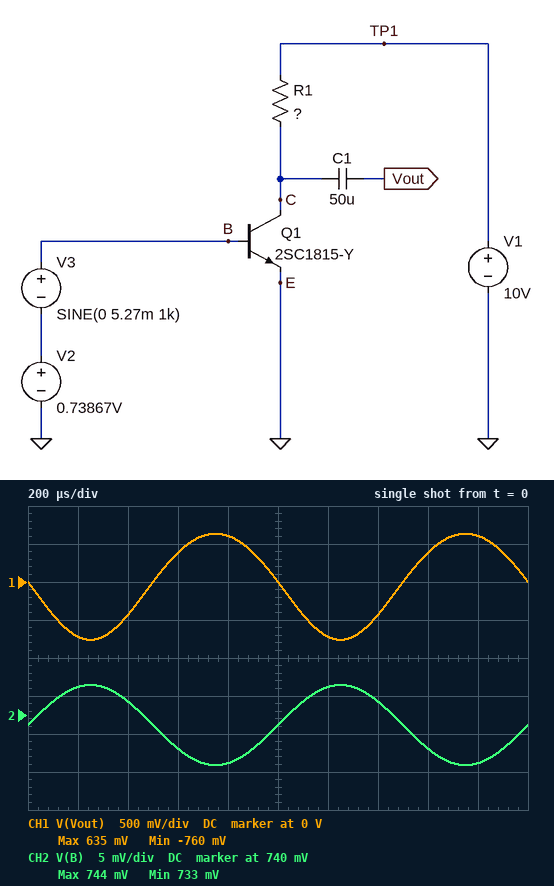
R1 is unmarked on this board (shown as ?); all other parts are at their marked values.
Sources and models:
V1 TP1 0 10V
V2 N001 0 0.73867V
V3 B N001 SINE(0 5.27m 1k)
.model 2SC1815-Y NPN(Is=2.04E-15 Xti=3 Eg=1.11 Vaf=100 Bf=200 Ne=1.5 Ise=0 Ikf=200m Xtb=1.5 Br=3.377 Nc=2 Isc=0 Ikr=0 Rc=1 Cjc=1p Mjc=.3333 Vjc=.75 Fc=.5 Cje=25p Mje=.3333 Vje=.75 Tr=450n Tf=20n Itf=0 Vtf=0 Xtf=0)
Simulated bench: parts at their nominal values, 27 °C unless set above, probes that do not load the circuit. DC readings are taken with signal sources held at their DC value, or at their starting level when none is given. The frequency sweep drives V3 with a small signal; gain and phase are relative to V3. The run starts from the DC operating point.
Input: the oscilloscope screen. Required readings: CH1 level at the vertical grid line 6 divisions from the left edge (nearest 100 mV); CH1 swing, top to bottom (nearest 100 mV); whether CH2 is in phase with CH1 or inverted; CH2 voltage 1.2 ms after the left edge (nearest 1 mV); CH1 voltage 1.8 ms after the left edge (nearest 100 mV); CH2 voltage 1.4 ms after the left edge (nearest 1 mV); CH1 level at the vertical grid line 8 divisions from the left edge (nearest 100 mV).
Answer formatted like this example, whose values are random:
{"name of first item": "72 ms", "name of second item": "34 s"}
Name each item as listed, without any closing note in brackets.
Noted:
{"CH1 level at the vertical grid line 6 divisions from the left edge": "-700 mV", "CH1 swing, top to bottom": "1.4 V", "whether CH2 is in phase with CH1 or inverted": "inverted", "CH2 voltage 1.2 ms after the left edge": "744 mV", "CH1 voltage 1.8 ms after the left edge": "600 mV", "CH2 voltage 1.4 ms after the left edge": "742 mV", "CH1 level at the vertical grid line 8 divisions from the left edge": "400 mV"}
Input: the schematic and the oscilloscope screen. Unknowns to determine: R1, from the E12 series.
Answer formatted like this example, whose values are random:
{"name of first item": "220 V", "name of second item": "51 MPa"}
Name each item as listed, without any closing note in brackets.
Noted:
{"R1, from the E12 series": "680 Ω"}
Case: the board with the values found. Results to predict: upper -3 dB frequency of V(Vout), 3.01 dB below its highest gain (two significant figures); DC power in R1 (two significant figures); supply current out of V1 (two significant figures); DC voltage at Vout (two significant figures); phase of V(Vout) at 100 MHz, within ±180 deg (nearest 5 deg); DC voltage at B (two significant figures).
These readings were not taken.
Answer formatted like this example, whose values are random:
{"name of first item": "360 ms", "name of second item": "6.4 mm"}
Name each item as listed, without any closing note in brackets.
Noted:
{"upper -3 dB frequency of V(Vout), 3.01 dB below its highest gain": "490 MHz", "DC power in R1": "19 mW", "supply current out of V1": "5.3 mA", "DC voltage at Vout": "6.4 V", "phase of V(Vout) at 100 MHz, within ±180 deg": "170 deg", "DC voltage at B": "740 mV"}
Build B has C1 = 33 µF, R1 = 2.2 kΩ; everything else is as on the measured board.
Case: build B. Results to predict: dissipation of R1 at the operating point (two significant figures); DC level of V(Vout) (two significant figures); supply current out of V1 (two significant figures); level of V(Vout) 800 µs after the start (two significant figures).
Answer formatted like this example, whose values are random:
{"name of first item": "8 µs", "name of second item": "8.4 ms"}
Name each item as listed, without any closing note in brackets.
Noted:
{"dissipation of R1 at the operating point": "45 mW", "DC level of V(Vout)": "72 mV", "supply current out of V1": "4.5 mA", "level of V(Vout) 800 µs after the start": "760 mV"}
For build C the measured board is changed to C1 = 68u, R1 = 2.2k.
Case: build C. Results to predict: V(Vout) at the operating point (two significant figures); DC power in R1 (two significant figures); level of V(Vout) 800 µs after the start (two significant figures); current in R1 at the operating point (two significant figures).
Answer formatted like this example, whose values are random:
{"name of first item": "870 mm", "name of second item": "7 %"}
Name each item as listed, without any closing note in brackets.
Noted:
{"V(Vout) at the operating point": "72 mV", "DC power in R1": "45 mW", "level of V(Vout) 800 µs after the start": "760 mV", "current in R1 at the operating point": "4.5 mA"}
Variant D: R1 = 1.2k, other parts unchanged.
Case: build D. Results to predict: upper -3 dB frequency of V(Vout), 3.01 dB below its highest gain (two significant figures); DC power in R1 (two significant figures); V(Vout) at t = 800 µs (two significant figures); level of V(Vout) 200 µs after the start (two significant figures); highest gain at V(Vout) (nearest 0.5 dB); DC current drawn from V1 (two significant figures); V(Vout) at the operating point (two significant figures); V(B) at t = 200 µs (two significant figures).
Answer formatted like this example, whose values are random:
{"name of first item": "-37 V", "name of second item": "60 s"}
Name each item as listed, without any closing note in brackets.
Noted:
{"upper -3 dB frequency of V(Vout), 3.01 dB below its highest gain": "240 MHz", "DC power in R1": "32 mW", "V(Vout) at t = 800 µs": "1.0 V", "level of V(Vout) 200 µs after the start": "-1.2 V", "highest gain at V(Vout)": "47.0 dB", "DC current drawn from V1": "5.2 mA", "V(Vout) at the operating point": "3.8 V", "V(B) at t = 200 µs": "740 mV"}
